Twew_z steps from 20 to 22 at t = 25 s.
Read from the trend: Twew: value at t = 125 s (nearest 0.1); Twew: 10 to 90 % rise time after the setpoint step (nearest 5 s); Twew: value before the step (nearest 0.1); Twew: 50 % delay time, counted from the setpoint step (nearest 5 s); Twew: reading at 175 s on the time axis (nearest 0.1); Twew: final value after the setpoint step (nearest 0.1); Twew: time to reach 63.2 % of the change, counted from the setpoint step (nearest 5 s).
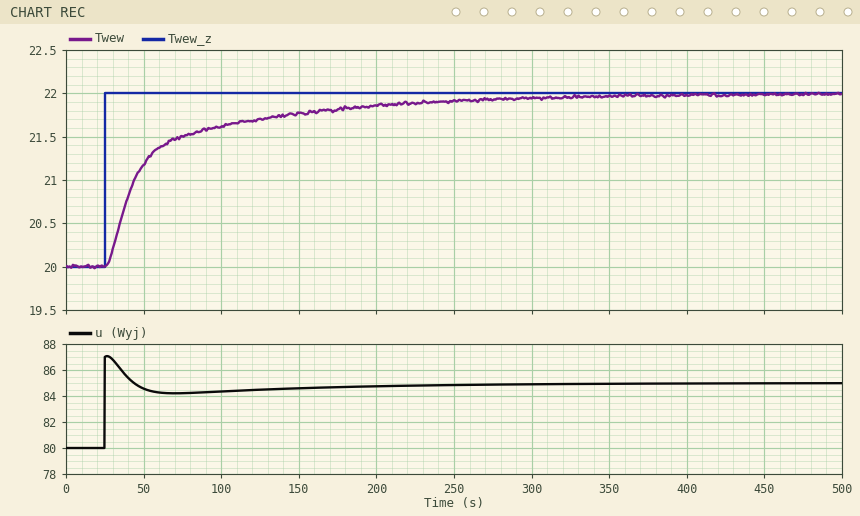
21.7
135 s
20.0
20 s
21.8
22.0
30 s
